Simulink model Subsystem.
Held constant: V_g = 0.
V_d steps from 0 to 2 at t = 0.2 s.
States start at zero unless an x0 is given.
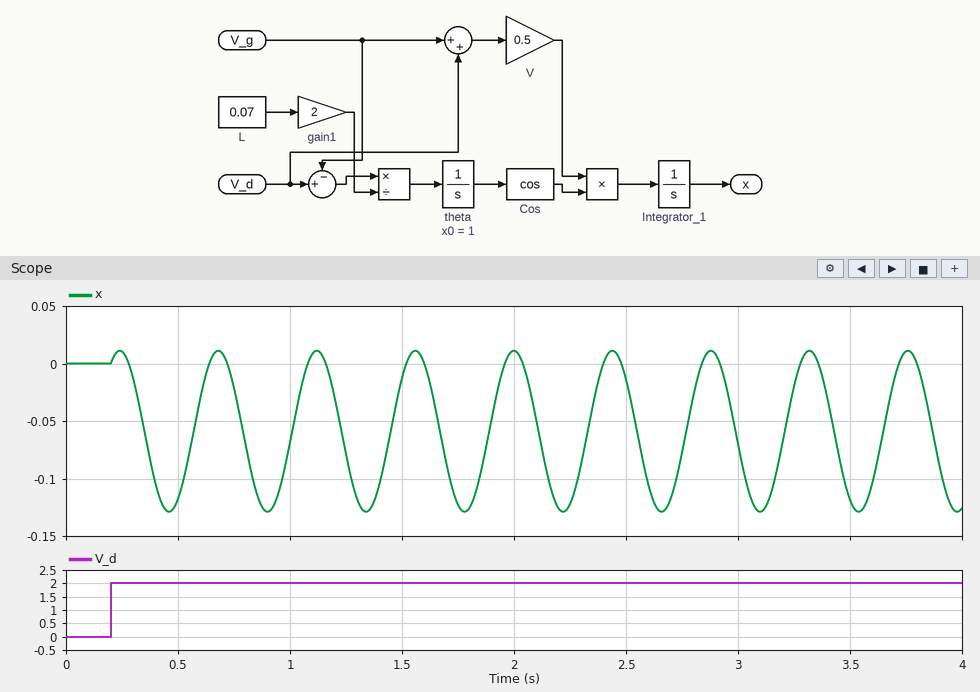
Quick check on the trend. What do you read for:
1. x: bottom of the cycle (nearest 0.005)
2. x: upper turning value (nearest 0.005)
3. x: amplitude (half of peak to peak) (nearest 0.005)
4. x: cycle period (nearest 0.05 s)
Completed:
-0.130
0.010
0.070
0.45 s
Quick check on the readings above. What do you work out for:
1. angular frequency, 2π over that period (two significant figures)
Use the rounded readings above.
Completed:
14 rad/s
